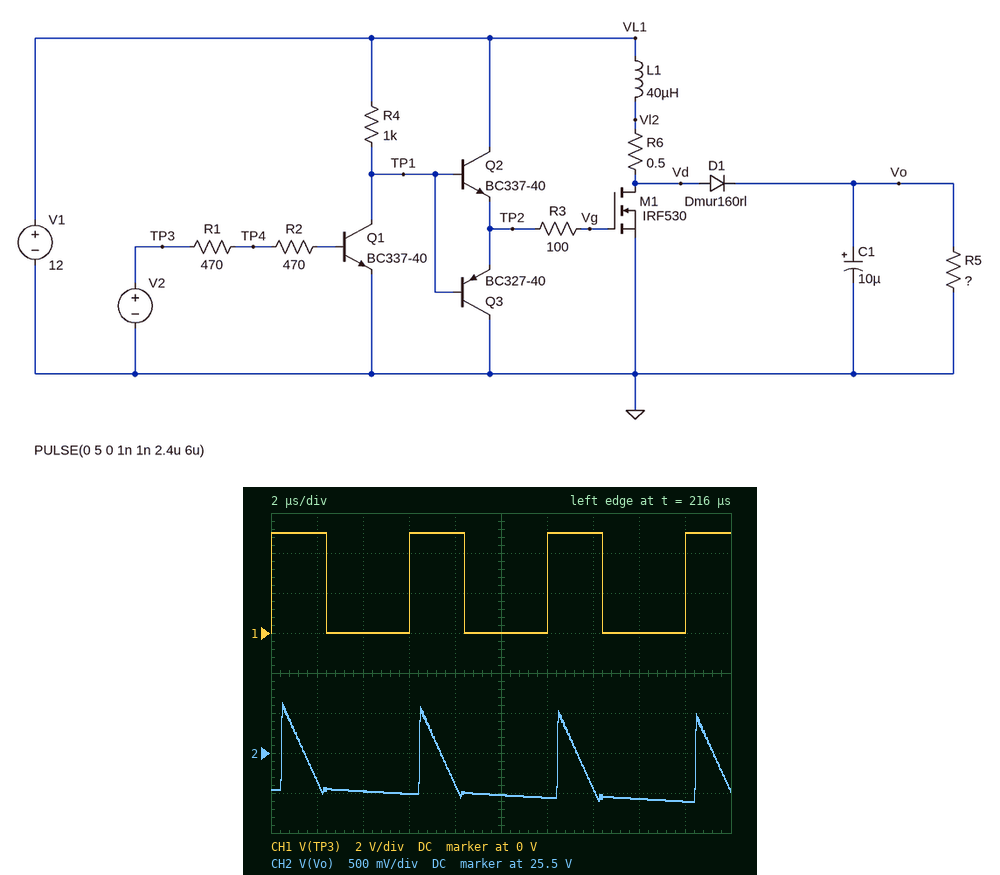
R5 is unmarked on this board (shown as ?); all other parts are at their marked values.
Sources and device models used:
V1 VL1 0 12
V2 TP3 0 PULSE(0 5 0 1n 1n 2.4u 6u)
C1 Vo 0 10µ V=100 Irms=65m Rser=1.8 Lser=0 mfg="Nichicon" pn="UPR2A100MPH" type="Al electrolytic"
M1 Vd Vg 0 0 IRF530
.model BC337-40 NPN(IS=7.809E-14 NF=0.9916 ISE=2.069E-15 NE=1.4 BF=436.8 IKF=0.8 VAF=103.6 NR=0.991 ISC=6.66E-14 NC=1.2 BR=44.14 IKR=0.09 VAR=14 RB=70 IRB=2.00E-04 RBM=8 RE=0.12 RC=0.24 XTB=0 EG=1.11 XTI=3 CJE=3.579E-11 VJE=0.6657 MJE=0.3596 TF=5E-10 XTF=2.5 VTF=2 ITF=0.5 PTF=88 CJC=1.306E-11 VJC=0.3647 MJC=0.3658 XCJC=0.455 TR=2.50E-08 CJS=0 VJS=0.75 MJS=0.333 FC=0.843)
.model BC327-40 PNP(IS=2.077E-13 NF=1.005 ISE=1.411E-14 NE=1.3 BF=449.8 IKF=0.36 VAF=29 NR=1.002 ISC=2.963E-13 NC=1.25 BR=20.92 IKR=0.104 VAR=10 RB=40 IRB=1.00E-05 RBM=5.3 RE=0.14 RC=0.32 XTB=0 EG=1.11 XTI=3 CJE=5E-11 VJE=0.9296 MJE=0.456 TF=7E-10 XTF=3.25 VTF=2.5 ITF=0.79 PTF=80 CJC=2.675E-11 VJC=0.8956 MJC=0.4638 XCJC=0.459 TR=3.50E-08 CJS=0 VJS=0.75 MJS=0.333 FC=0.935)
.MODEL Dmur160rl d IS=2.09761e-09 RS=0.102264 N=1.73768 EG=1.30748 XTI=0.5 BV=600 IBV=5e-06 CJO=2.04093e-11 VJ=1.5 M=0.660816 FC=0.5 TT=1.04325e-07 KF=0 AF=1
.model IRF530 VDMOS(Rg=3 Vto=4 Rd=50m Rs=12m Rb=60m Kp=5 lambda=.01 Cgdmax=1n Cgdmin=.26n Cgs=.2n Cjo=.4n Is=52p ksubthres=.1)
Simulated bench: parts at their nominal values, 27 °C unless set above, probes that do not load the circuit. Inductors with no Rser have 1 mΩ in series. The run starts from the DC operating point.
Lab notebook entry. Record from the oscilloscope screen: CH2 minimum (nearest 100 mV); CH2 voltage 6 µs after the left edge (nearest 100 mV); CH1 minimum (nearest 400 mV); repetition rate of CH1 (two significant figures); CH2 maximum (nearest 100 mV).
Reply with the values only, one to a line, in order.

24.9 V
25.0 V
0 V
170 kHz
26.1 V
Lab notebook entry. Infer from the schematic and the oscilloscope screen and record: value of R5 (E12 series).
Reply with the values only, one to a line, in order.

150 Ω
